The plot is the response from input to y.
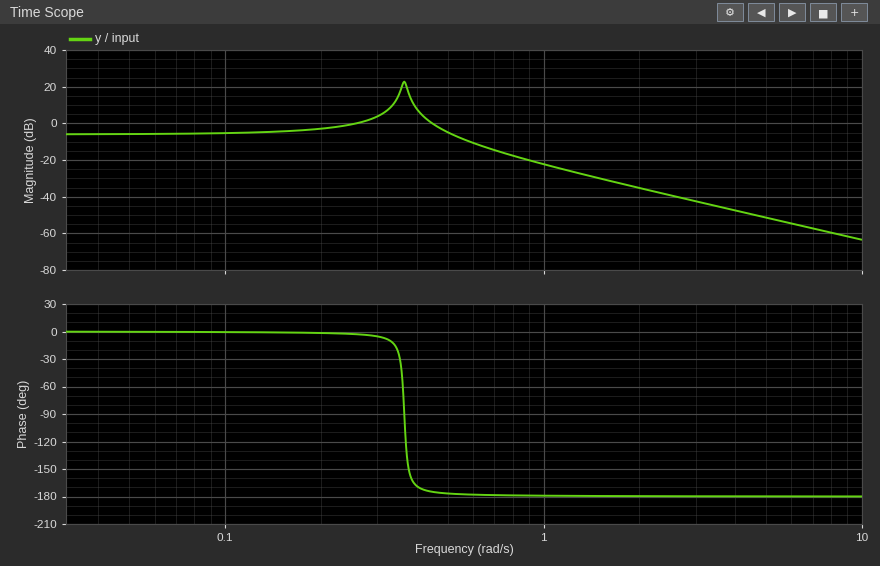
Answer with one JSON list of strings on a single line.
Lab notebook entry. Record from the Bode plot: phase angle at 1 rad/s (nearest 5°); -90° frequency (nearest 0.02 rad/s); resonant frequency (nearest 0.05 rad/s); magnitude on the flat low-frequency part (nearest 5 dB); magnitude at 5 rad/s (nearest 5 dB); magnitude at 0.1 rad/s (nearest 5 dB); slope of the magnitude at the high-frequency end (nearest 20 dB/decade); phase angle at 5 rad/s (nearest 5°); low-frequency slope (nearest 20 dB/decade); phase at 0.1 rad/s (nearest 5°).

["-180°", "0.36 rad/s", "0.35 rad/s", "-5 dB", "-50 dB", "-5 dB", "-40 dB/decade", "-180°", "0 dB/decade", "0°"]
